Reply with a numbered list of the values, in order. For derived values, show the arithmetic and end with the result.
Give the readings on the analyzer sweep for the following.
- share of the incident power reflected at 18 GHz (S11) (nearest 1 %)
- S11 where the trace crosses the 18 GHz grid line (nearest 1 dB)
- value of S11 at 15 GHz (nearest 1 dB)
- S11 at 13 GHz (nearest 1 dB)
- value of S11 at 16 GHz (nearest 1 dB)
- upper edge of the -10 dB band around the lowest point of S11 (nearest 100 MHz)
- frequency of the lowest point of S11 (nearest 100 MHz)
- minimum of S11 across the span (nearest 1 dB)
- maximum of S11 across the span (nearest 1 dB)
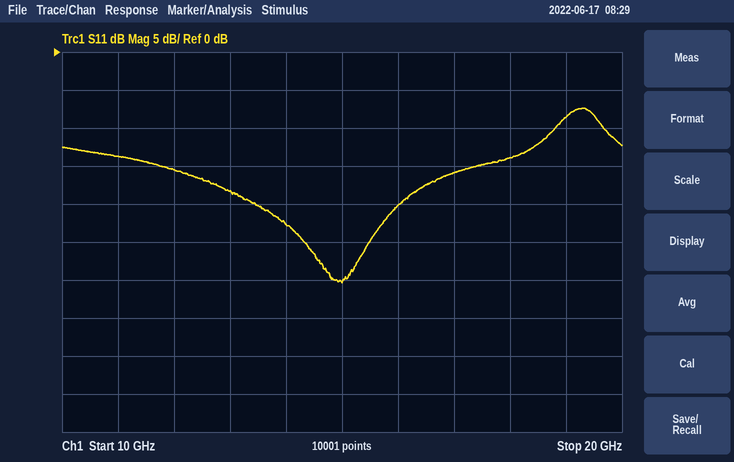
1. 10^(-14/10) ≈ 4 %
2. -14 dB
3. -30 dB
4. -18 dB
5. -20 dB
6. 18.8 GHz
7. 15.0 GHz
8. -30 dB
9. -7 dB
